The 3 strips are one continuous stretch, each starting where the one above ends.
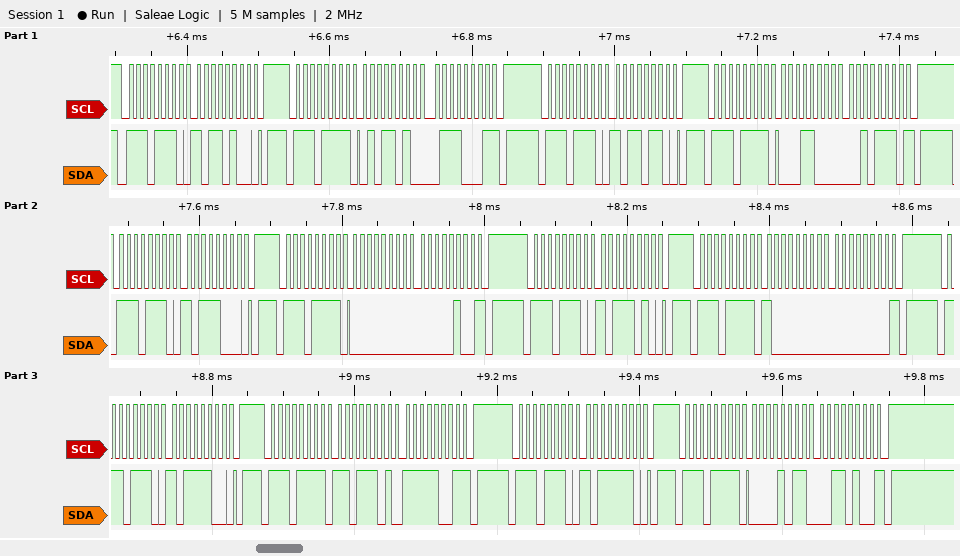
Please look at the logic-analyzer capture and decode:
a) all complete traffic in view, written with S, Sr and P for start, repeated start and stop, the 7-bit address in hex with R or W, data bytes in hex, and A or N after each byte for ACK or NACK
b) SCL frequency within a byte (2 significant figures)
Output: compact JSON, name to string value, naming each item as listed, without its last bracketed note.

{"all complete traffic in view, written with S, Sr and P for start, repeated start and stop, the 7-bit address in hex with R or W, data bytes in hex, and A or N after each byte for ACK or NACK": "S 77W A B4 A P S 77R A 5A A 71 N P S 77W A B6 A P S 77R A 18 A 2E N P S 77W A B8 A P S 77R A 00 A 04 N P S 77W A BA A P S 77R A 80 A 00 N P S 77W A BC A P S 77R A DD A F9 N P S 77W A BE A P S 77R A 0B A 34 N P", "SCL frequency within a byte": "100 kHz"}
